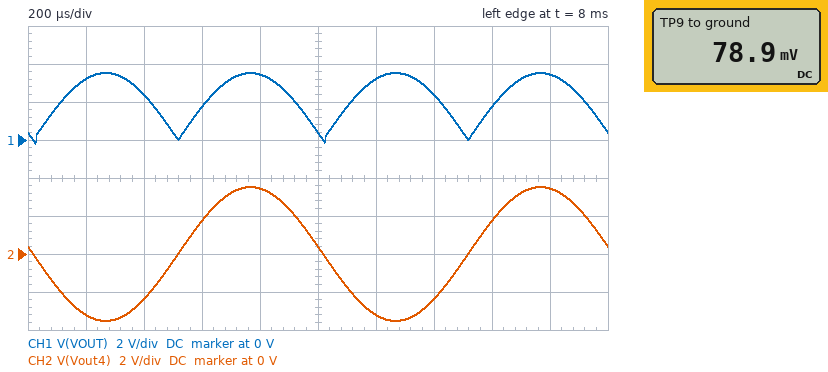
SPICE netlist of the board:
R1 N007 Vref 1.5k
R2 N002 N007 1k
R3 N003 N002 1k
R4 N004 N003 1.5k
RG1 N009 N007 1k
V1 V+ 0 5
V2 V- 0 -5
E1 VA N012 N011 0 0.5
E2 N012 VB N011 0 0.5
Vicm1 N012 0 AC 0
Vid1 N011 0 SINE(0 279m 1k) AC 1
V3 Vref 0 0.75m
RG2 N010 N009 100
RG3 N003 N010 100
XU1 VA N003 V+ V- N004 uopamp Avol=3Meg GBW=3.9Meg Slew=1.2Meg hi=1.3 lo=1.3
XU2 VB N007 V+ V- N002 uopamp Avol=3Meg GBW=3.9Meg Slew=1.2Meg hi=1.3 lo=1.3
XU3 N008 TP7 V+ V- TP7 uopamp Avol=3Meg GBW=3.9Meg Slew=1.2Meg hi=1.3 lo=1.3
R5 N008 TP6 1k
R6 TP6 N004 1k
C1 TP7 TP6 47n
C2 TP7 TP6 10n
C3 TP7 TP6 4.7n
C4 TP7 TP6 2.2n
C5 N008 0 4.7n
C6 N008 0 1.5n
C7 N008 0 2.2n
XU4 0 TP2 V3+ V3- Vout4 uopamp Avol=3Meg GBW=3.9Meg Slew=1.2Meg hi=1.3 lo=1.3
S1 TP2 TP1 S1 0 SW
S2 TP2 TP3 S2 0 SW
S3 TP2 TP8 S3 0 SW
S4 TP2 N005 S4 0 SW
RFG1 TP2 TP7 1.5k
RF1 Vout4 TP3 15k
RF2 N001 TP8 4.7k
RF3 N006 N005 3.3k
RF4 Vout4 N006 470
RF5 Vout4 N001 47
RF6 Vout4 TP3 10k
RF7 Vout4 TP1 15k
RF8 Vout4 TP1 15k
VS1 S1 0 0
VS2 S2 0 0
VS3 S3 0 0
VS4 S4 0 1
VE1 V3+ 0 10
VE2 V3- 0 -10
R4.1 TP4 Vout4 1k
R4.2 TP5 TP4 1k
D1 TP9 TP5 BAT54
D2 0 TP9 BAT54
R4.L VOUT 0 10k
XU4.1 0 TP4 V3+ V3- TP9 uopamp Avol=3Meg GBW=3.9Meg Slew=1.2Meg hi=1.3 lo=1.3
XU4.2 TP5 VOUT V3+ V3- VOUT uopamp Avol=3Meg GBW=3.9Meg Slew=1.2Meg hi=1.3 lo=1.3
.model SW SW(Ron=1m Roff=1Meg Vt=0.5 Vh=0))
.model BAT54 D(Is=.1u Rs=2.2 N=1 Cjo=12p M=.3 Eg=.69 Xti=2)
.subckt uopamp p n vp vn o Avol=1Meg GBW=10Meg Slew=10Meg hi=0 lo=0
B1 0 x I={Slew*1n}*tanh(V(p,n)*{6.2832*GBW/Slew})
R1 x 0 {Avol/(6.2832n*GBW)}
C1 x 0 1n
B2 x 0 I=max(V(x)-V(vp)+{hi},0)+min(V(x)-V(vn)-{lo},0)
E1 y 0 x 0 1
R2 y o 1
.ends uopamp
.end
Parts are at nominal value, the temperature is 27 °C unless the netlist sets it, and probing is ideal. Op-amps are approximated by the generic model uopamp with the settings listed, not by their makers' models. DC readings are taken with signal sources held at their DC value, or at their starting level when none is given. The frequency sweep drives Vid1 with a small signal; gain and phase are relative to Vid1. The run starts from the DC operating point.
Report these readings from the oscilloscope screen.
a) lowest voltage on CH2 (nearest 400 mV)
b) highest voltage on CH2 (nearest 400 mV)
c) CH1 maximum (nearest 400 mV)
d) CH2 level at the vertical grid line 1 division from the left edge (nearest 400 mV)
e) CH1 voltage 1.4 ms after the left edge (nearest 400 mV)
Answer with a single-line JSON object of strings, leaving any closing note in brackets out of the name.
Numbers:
{"lowest voltage on CH2": "-3.6 V", "highest voltage on CH2": "3.6 V", "CH1 maximum": "3.6 V", "CH2 level at the vertical grid line 1 division from the left edge": "-3.2 V", "CH1 voltage 1.4 ms after the left edge": "2.4 V"}
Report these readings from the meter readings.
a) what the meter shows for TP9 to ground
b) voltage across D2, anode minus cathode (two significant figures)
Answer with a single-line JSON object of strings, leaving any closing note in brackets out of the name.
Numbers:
{"what the meter shows for TP9 to ground": "78.9 mV", "voltage across D2, anode minus cathode": "-79 mV"}
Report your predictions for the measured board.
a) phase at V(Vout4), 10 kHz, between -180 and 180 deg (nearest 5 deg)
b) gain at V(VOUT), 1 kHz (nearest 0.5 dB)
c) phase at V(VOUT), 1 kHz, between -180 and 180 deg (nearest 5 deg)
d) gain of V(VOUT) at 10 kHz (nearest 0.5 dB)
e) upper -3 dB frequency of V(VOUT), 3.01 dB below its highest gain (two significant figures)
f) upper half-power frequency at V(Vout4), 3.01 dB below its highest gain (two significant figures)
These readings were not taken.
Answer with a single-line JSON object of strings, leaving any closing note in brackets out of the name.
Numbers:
{"phase at V(Vout4), 10 kHz, between -180 and 180 deg": "20 deg", "gain at V(VOUT), 1 kHz": "58.5 dB", "phase at V(VOUT), 1 kHz, between -180 and 180 deg": "-10 deg", "gain of V(VOUT) at 10 kHz": "54.0 dB", "upper -3 dB frequency of V(VOUT), 3.01 dB below its highest gain": "8.0 kHz", "upper half-power frequency at V(Vout4), 3.01 dB below its highest gain": "8.0 kHz"}
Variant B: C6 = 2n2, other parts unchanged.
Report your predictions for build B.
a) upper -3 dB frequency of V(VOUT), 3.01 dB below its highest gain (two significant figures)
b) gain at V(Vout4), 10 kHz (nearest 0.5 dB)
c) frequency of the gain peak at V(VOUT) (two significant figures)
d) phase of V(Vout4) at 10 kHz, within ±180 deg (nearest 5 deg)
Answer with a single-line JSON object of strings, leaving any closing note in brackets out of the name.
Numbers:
{"upper -3 dB frequency of V(VOUT), 3.01 dB below its highest gain": "7.7 kHz", "gain at V(Vout4), 10 kHz": "53.0 dB", "frequency of the gain peak at V(VOUT)": "5.5 kHz", "phase of V(Vout4) at 10 kHz, within ±180 deg": "15 deg"}
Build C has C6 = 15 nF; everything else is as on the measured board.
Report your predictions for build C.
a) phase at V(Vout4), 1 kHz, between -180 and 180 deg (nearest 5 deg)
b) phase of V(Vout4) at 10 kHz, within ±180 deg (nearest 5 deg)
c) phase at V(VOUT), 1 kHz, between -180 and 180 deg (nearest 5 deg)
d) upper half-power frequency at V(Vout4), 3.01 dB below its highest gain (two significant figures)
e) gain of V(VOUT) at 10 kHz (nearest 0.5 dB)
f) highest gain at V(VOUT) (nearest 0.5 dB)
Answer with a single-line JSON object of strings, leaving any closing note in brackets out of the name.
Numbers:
{"phase at V(Vout4), 1 kHz, between -180 and 180 deg": "160 deg", "phase of V(Vout4) at 10 kHz, within ±180 deg": "5 deg", "phase at V(VOUT), 1 kHz, between -180 and 180 deg": "-20 deg", "upper half-power frequency at V(Vout4), 3.01 dB below its highest gain": "4.7 kHz", "gain of V(VOUT) at 10 kHz": "43.0 dB", "highest gain at V(VOUT)": "59.0 dB"}
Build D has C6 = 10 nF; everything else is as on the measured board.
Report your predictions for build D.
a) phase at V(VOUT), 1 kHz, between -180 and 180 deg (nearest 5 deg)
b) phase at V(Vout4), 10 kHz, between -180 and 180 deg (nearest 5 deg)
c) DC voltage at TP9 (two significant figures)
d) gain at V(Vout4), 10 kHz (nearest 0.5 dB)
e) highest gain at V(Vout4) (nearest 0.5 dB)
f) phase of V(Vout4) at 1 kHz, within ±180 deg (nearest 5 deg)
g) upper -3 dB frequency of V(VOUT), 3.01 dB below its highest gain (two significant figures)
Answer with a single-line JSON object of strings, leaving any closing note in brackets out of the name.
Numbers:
{"phase at V(VOUT), 1 kHz, between -180 and 180 deg": "-15 deg", "phase at V(Vout4), 10 kHz, between -180 and 180 deg": "10 deg", "DC voltage at TP9": "79 mV", "gain at V(Vout4), 10 kHz": "46.0 dB", "highest gain at V(Vout4)": "59.5 dB", "phase of V(Vout4) at 1 kHz, within ±180 deg": "165 deg", "upper -3 dB frequency of V(VOUT), 3.01 dB below its highest gain": "5.6 kHz"}
